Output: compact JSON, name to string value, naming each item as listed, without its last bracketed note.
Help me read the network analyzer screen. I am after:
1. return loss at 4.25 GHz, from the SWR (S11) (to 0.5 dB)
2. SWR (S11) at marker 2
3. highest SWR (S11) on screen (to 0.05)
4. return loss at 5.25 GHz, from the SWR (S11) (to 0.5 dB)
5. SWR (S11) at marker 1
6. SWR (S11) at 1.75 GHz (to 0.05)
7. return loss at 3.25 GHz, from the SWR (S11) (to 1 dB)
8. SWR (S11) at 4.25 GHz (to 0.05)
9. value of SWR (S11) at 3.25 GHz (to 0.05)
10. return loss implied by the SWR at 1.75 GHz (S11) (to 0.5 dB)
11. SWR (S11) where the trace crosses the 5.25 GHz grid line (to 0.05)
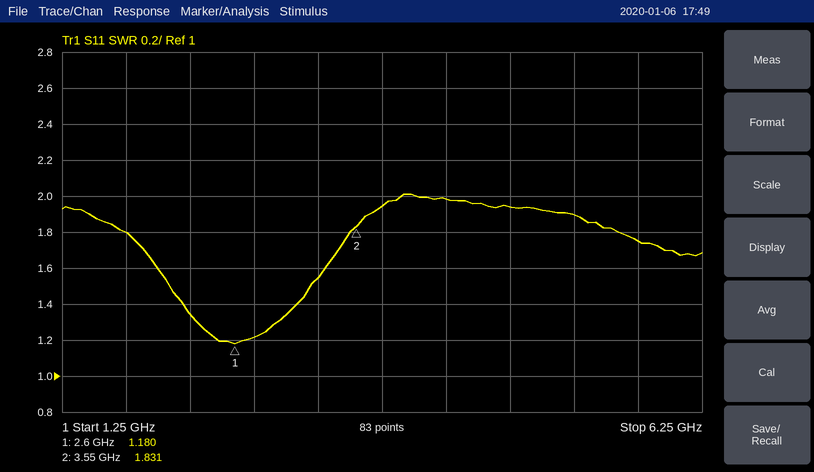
{"return loss at 4.25 GHz, from the SWR (S11)": "9.5 dB", "SWR (S11) at marker 2": "1.831", "highest SWR (S11) on screen": "2.00", "return loss at 5.25 GHz, from the SWR (S11)": "10.0 dB", "SWR (S11) at marker 1": "1.180", "SWR (S11) at 1.75 GHz": "1.80", "return loss at 3.25 GHz, from the SWR (S11)": "13 dB", "SWR (S11) at 4.25 GHz": "2.00", "value of SWR (S11) at 3.25 GHz": "1.55", "return loss implied by the SWR at 1.75 GHz (S11)": "11.0 dB", "SWR (S11) where the trace crosses the 5.25 GHz grid line": "1.90"}
